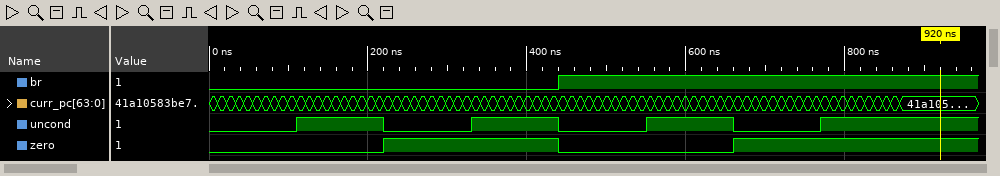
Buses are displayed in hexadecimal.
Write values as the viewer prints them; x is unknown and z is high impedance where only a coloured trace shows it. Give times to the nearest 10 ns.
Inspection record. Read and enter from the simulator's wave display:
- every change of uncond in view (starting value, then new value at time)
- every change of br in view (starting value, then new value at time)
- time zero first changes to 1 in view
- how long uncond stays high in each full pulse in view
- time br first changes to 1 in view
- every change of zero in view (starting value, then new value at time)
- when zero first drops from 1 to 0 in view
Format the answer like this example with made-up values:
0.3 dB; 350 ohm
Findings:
0, 1 at 110 ns, 0 at 220 ns, 1 at 330 ns, 0 at 440 ns, 1 at 550 ns, 0 at 660 ns, 1 at 770 ns; 0, 1 at 440 ns; 220 ns; 110 ns, 110 ns, 110 ns; 440 ns; 0, 1 at 220 ns, 0 at 440 ns, 1 at 660 ns; 440 ns
